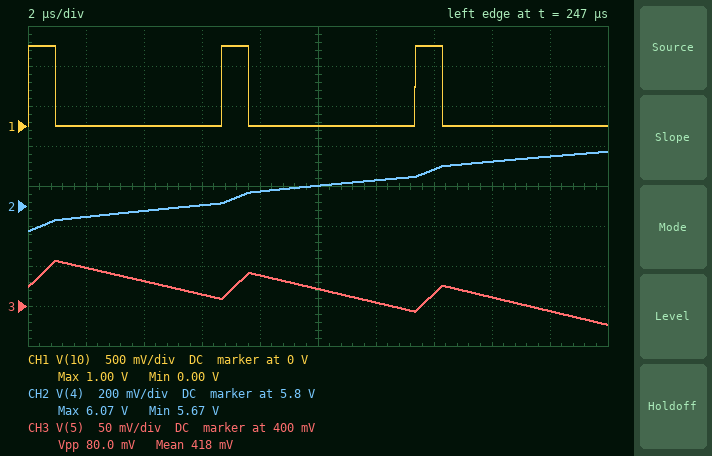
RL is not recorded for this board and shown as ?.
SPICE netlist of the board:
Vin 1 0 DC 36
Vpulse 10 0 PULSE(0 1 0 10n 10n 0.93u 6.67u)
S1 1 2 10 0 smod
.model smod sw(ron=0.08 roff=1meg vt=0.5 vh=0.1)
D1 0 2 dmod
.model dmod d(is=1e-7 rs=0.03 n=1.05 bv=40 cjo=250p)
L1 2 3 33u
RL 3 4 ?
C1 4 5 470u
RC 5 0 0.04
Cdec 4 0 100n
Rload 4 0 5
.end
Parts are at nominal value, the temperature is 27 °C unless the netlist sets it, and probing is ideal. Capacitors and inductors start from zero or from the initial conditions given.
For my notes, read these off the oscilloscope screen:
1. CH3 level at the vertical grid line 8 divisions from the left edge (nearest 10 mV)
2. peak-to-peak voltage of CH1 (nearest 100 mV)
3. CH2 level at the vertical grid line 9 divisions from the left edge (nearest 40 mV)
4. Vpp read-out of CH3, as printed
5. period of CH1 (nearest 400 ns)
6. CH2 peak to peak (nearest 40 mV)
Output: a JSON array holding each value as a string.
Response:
["410 mV", "1.0 V", "6.04 V", "80.0 mV", "6.8 µs", "400 mV"]
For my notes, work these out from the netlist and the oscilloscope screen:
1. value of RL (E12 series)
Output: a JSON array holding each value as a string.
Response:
["0.012 Ω"]
